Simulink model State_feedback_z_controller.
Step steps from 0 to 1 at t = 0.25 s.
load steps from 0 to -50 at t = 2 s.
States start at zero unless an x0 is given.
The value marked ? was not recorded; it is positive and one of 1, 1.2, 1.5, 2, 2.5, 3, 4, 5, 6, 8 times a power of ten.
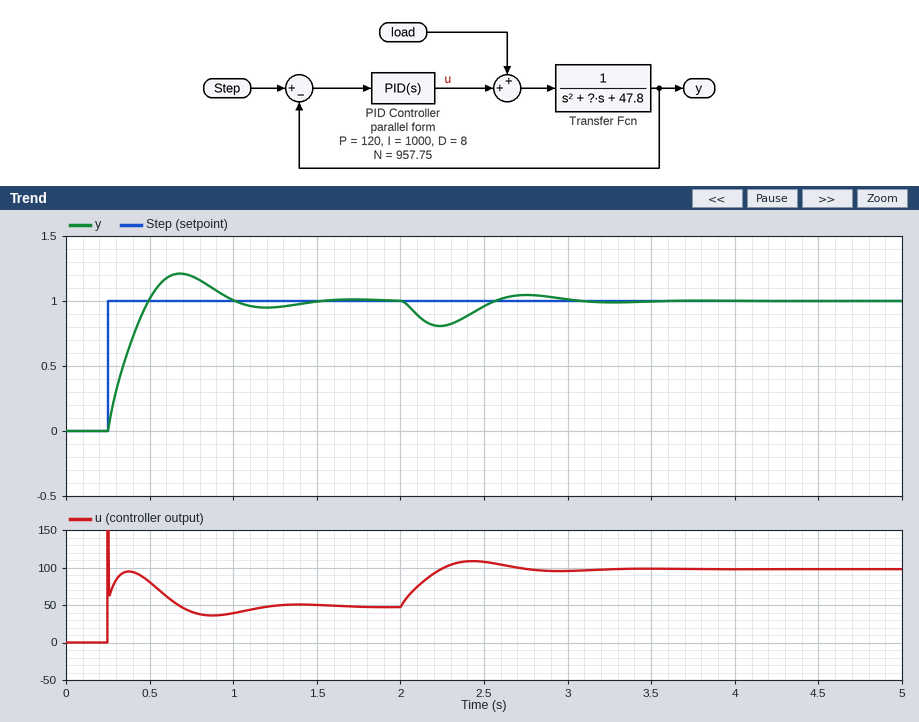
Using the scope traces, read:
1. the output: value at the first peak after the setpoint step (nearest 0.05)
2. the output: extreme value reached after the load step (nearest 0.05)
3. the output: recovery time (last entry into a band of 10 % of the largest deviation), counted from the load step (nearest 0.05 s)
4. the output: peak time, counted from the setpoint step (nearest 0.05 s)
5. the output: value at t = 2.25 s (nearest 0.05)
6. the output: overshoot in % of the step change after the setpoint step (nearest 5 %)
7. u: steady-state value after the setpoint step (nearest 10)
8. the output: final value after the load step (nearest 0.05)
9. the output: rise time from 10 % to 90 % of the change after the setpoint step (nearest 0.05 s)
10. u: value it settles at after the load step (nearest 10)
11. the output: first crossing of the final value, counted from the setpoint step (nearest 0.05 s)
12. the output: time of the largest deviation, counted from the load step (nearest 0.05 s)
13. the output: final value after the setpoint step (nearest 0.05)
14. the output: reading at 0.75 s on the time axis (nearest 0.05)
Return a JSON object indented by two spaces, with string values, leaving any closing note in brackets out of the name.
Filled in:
{
  "the output: value at the first peak after the setpoint step": "1.20",
  "the output: extreme value reached after the load step": "0.80",
  "the output: recovery time (last entry into a band of 10 % of the largest deviation), counted from the load step": "0.95 s",
  "the output: peak time, counted from the setpoint step": "0.45 s",
  "the output: value at t = 2.25 s": "0.80",
  "the output: overshoot in % of the step change after the setpoint step": "20 %",
  "u: steady-state value after the setpoint step": "50",
  "the output: final value after the load step": "1.00",
  "the output: rise time from 10 % to 90 % of the change after the setpoint step": "0.20 s",
  "u: value it settles at after the load step": "100",
  "the output: first crossing of the final value, counted from the setpoint step": "0.25 s",
  "the output: time of the largest deviation, counted from the load step": "0.25 s",
  "the output: final value after the setpoint step": "1.00",
  "the output: reading at 0.75 s on the time axis": "1.20"
}
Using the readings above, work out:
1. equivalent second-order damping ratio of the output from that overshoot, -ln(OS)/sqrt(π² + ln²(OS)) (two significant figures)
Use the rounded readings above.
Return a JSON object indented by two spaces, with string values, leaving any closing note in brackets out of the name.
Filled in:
{
  "equivalent second-order damping ratio of the output from that overshoot, -ln(OS)/sqrt(π² + ln²(OS))": "0.46"
}
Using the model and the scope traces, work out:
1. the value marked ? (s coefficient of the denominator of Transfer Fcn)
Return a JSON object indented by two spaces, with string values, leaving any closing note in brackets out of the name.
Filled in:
{
  "the value marked ?": "20"
}
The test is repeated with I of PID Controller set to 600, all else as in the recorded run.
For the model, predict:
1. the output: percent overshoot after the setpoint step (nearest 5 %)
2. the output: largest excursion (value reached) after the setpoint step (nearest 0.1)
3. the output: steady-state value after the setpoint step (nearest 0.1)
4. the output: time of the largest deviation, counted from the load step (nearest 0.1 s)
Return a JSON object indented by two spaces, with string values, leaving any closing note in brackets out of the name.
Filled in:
{
  "the output: percent overshoot after the setpoint step": "10 %",
  "the output: largest excursion (value reached) after the setpoint step": "1.1",
  "the output: steady-state value after the setpoint step": "1.0",
  "the output: time of the largest deviation, counted from the load step": "0.3 s"
}
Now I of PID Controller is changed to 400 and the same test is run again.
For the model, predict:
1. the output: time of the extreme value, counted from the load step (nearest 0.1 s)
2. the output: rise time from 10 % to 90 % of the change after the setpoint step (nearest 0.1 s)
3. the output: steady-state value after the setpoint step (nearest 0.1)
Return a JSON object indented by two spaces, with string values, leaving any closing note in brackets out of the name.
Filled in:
{
  "the output: time of the extreme value, counted from the load step": "0.3 s",
  "the output: rise time from 10 % to 90 % of the change after the setpoint step": "0.3 s",
  "the output: steady-state value after the setpoint step": "1.0"
}
